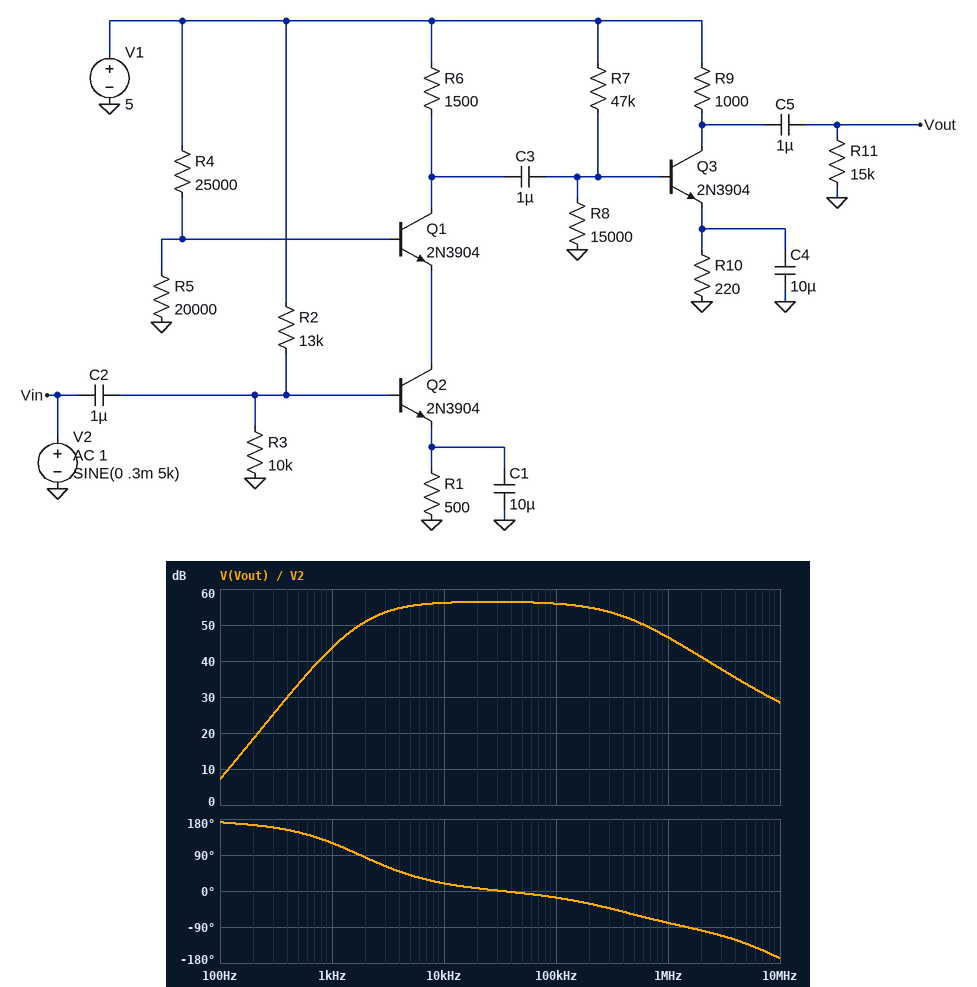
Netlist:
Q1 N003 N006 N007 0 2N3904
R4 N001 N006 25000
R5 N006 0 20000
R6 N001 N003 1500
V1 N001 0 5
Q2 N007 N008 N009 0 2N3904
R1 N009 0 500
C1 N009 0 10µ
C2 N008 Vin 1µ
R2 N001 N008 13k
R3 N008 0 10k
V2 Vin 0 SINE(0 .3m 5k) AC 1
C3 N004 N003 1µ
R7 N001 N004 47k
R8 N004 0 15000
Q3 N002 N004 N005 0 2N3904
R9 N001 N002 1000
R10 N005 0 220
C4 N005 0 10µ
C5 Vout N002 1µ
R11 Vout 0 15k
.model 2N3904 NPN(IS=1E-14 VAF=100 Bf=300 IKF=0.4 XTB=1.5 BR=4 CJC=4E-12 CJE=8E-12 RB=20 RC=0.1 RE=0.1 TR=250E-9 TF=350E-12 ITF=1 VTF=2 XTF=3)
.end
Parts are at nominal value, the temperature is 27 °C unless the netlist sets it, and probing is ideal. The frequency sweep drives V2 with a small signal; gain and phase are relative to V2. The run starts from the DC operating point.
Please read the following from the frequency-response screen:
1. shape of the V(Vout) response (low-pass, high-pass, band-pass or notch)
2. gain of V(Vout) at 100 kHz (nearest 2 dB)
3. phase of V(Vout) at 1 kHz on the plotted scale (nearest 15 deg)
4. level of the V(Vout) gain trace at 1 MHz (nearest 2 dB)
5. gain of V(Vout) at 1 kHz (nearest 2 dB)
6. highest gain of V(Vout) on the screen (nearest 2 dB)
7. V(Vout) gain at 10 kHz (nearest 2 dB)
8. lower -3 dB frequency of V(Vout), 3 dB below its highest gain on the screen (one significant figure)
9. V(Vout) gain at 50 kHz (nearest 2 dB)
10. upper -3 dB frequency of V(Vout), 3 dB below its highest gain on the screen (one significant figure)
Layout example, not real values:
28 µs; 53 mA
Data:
band-pass; 56 dB; 120 deg; 46 dB; 44 dB; 56 dB; 56 dB; 3 kHz; 56 dB; 300 kHz
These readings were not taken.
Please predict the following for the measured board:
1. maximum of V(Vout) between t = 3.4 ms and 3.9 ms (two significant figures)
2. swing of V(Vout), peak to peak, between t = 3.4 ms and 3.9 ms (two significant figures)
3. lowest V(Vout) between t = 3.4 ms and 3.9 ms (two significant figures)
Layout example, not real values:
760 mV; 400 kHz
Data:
170 mV; 350 mV; -180 mV
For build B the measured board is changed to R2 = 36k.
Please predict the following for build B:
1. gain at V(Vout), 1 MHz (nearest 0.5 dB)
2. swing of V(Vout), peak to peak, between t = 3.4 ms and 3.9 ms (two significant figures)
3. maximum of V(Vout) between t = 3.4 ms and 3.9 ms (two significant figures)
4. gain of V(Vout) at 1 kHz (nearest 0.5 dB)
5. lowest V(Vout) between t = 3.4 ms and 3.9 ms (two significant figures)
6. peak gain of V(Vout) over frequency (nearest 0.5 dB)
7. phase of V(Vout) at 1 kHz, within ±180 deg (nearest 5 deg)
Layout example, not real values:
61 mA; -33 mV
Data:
62.0 dB; 1.3 V; 610 mV; 63.0 dB; -690 mV; 67.0 dB; 70 deg
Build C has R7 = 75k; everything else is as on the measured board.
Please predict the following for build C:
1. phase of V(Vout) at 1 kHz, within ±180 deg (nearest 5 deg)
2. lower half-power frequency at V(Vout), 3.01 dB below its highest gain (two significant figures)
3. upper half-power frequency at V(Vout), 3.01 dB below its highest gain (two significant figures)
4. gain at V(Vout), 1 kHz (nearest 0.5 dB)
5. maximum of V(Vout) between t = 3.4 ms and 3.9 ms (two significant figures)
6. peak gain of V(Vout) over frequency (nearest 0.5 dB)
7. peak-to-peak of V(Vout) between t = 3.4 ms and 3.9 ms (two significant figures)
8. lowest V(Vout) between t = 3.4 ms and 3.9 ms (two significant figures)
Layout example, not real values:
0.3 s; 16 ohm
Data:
95 deg; 2.5 kHz; 320 kHz; 38.0 dB; 62 mV; 47.5 dB; 130 mV; -68 mV
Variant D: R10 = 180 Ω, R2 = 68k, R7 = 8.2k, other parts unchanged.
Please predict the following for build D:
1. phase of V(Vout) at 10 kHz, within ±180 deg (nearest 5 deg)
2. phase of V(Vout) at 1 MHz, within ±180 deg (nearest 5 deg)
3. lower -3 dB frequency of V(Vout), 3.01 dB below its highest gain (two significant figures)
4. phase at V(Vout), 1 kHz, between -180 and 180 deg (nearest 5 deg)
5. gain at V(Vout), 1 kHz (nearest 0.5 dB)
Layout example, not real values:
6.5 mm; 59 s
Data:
0 deg; -110 deg; 100 Hz; 25 deg; -14.0 dB
